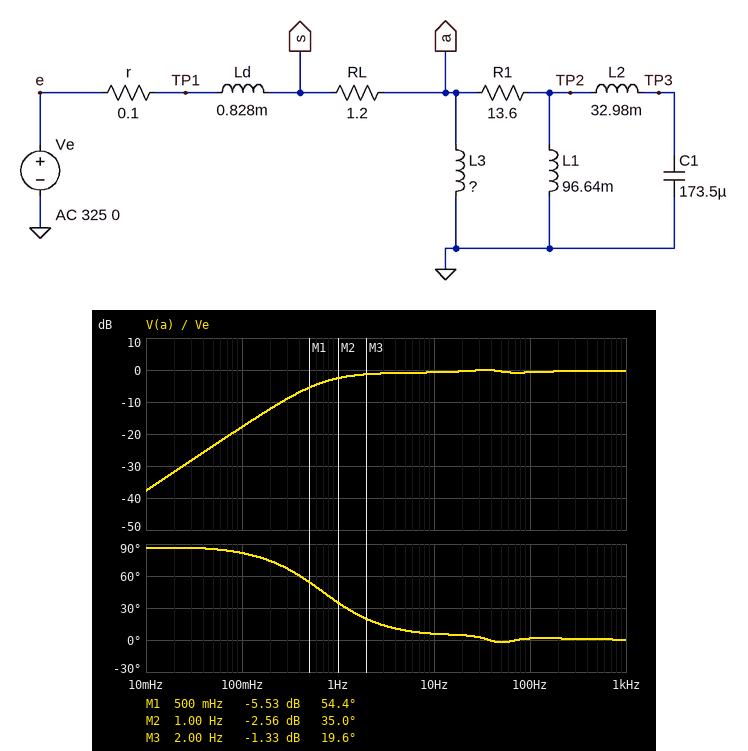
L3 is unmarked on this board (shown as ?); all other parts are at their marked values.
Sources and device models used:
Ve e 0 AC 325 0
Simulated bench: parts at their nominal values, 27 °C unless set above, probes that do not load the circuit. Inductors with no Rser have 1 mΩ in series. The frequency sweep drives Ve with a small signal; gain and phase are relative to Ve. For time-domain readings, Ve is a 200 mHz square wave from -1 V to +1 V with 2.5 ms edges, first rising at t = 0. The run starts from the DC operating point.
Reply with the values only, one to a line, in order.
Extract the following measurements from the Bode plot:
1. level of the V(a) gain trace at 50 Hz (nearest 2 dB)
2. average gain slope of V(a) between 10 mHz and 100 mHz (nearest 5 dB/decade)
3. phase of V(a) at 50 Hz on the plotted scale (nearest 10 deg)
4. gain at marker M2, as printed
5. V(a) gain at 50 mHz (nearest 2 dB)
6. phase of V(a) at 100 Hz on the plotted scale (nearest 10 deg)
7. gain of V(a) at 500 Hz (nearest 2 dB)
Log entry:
0 dB
20 dB/decade
0 deg
-2.56 dB
-24 dB
0 deg
0 dB
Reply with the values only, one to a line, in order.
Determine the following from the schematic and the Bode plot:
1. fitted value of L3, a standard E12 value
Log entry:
270 mH
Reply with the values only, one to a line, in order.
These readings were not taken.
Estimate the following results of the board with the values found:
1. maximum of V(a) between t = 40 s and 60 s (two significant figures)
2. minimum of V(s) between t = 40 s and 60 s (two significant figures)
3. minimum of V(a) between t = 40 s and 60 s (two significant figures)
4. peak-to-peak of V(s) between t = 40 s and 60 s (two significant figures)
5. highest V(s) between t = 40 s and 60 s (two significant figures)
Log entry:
1.9 V
-1.1 V
-1.9 V
2.1 V
1.1 V
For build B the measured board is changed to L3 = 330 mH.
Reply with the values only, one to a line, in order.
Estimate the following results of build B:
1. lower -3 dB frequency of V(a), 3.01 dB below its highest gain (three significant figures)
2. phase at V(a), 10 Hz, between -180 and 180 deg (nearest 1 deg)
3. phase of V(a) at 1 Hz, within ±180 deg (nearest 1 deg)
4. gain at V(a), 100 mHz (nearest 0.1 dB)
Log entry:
703 mHz
5 deg
30 deg
-16.1 dB
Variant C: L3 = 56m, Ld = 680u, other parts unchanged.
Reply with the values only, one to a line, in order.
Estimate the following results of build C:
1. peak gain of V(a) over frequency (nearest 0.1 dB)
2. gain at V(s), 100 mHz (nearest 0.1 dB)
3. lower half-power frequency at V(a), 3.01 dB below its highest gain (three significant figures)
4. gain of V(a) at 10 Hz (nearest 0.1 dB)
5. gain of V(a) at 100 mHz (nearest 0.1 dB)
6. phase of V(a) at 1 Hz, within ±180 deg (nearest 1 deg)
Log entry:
-0.1 dB
-0.7 dB
4.10 Hz
-1.3 dB
-31.4 dB
73 deg
